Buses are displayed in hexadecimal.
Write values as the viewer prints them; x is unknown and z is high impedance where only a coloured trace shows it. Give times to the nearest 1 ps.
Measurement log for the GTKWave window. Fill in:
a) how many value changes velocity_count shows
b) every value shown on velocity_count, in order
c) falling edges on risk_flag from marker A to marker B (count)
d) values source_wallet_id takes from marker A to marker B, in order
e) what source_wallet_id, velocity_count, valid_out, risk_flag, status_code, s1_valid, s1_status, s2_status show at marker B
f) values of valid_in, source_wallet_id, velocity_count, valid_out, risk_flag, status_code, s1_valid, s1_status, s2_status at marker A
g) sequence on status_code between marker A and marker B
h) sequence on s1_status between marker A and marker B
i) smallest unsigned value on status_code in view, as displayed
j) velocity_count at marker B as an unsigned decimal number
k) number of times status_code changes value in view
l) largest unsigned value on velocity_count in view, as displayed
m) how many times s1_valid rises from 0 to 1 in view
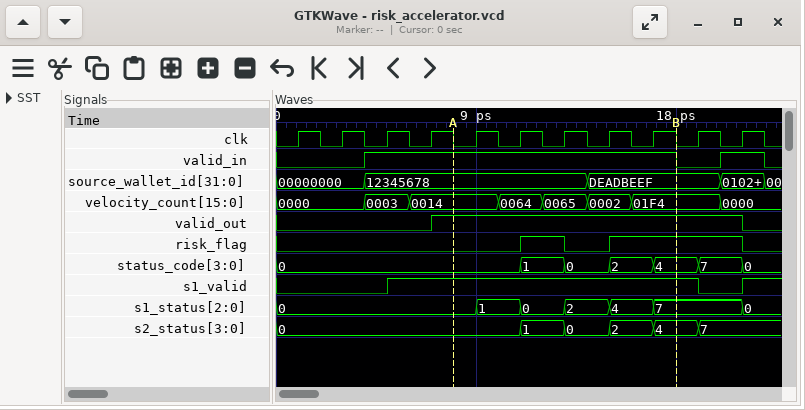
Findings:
7
0000, 0003, 0014, 0064, 0065, 0002, 01F4, 0000
1
12345678, DEADBEEF
source_wallet_id=DEADBEEF, velocity_count=01F4, valid_out=1, risk_flag=1, status_code=4, s1_valid=1, s1_status=7, s2_status=4
valid_in=1, source_wallet_id=12345678, velocity_count=0014, valid_out=1, risk_flag=0, status_code=0, s1_valid=1, s1_status=0, s2_status=0
0, 1, 0, 2, 4
0, 1, 0, 2, 4, 7
0
500
6
01F4
2
